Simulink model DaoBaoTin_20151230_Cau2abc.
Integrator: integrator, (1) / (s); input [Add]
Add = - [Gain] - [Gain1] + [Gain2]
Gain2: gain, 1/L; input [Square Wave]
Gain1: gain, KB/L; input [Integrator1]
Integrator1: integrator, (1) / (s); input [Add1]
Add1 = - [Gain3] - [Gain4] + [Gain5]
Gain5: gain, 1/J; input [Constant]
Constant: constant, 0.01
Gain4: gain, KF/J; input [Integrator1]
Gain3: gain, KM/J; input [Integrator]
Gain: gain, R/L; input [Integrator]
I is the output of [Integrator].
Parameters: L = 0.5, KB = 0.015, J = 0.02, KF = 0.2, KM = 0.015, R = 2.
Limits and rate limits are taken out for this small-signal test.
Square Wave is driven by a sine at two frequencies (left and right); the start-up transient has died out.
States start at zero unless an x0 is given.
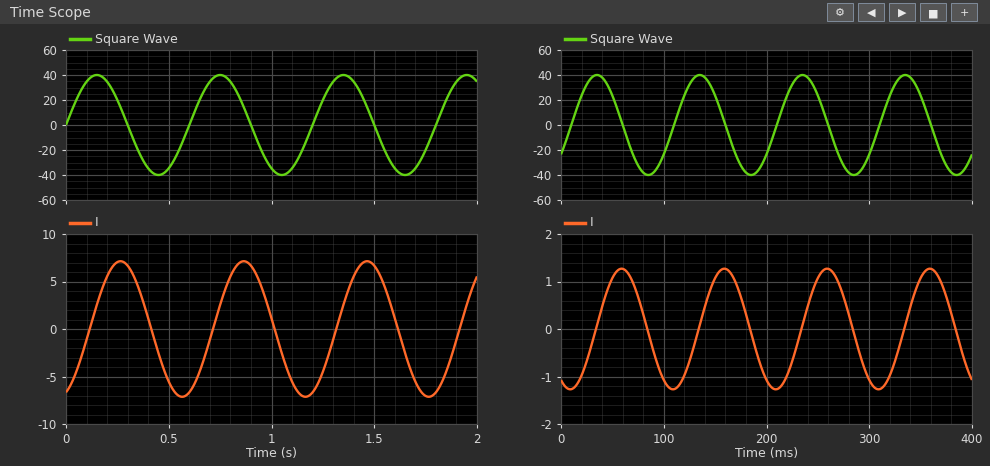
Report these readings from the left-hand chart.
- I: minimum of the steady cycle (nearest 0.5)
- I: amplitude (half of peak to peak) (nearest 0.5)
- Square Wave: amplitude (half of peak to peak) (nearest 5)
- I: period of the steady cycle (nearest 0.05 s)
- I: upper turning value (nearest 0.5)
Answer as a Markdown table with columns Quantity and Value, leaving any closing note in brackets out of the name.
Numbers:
| Quantity | Value |
|---|---|
| I: minimum of the steady cycle | -7.0 |
| I: amplitude (half of peak to peak) | 7.0 |
| Square Wave: amplitude (half of peak to peak) | 40 |
| I: period of the steady cycle | 0.60 s |
| I: upper turning value | 7.0 |
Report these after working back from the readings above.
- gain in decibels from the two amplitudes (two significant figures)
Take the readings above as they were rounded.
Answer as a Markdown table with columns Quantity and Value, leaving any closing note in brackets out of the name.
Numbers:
| Quantity | Value |
|---|---|
| gain in decibels from the two amplitudes | -15 dB |
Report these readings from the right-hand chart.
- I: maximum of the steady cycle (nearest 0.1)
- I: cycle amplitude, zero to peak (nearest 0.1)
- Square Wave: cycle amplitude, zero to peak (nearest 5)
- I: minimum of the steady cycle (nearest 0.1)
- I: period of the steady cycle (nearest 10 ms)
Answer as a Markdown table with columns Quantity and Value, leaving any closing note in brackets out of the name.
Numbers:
| Quantity | Value |
|---|---|
| I: maximum of the steady cycle | 1.3 |
| I: cycle amplitude, zero to peak | 1.3 |
| Square Wave: cycle amplitude, zero to peak | 40 |
| I: minimum of the steady cycle | -1.3 |
| I: period of the steady cycle | 100 ms |
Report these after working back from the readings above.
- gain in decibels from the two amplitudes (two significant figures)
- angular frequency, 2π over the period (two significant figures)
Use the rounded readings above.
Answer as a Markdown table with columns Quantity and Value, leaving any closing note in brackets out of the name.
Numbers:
| Quantity | Value |
|---|---|
| gain in decibels from the two amplitudes | -30 dB |
| angular frequency, 2π over the period | 0.063 rad/ms |
